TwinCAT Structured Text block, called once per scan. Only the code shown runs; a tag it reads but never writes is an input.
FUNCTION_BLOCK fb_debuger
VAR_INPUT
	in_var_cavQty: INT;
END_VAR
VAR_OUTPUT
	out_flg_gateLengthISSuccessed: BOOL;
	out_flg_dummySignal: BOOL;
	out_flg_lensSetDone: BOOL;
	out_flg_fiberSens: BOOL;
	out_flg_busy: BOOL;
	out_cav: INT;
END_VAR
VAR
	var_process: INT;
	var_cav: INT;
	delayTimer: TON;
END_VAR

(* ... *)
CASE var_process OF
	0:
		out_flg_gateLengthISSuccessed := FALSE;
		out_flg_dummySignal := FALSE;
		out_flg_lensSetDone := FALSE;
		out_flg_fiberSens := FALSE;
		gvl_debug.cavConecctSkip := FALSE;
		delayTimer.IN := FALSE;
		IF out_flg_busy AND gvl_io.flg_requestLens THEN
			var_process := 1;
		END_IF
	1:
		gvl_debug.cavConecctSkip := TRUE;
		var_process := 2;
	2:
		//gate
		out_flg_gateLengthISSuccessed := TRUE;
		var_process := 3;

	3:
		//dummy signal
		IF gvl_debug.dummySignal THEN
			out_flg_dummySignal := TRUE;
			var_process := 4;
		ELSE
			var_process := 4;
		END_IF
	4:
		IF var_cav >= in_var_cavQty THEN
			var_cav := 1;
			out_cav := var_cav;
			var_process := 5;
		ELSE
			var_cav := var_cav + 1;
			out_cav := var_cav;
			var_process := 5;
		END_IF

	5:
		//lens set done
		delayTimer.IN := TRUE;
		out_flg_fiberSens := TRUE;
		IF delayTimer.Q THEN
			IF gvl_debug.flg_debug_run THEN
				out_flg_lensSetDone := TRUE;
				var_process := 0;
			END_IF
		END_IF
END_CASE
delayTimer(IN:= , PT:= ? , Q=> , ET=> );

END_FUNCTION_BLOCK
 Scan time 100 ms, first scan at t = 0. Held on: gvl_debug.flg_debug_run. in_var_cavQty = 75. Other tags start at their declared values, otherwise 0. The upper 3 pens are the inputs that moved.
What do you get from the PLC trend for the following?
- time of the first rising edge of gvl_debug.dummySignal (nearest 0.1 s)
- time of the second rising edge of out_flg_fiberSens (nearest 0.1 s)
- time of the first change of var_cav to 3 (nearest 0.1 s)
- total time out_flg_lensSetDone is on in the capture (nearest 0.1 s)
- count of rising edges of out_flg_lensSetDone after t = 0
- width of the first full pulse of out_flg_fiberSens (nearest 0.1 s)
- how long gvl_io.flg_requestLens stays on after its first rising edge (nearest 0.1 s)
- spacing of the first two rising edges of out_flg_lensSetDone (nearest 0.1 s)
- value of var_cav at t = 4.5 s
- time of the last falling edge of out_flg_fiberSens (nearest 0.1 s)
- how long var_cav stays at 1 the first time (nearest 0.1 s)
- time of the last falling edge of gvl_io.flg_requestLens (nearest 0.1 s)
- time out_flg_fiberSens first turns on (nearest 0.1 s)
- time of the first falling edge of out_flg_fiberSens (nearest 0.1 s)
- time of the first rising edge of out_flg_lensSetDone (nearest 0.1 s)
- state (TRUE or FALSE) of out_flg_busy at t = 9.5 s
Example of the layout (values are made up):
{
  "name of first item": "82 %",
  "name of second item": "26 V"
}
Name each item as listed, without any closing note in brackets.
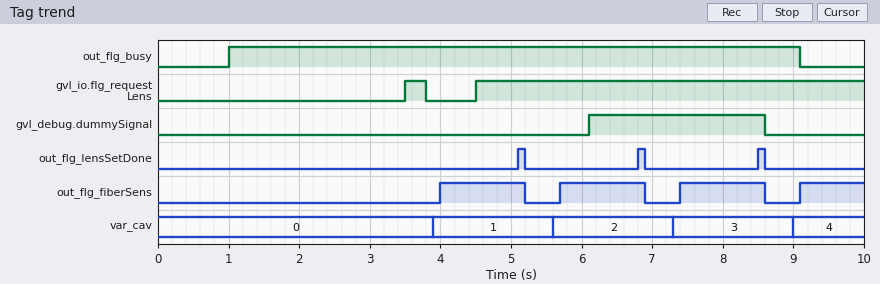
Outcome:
{
  "time of the first rising edge of gvl_debug.dummySignal": "6.1 s",
  "time of the second rising edge of out_flg_fiberSens": "5.7 s",
  "time of the first change of var_cav to 3": "7.3 s",
  "total time out_flg_lensSetDone is on in the capture": "0.3 s",
  "count of rising edges of out_flg_lensSetDone after t = 0": "3",
  "width of the first full pulse of out_flg_fiberSens": "1.2 s",
  "how long gvl_io.flg_requestLens stays on after its first rising edge": "0.3 s",
  "spacing of the first two rising edges of out_flg_lensSetDone": "1.7 s",
  "value of var_cav at t = 4.5 s": "1",
  "time of the last falling edge of out_flg_fiberSens": "8.6 s",
  "how long var_cav stays at 1 the first time": "1.7 s",
  "time of the last falling edge of gvl_io.flg_requestLens": "3.8 s",
  "time out_flg_fiberSens first turns on": "4.0 s",
  "time of the first falling edge of out_flg_fiberSens": "5.2 s",
  "time of the first rising edge of out_flg_lensSetDone": "5.1 s",
  "state (TRUE or FALSE) of out_flg_busy at t = 9.5 s": "FALSE"
}
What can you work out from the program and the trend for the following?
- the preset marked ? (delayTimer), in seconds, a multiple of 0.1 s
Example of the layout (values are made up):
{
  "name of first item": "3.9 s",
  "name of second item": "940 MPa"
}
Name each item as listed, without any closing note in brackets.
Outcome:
{
  "the preset marked ? (delayTimer), in seconds, a multiple of 0.1 s": "1.0 s"
}
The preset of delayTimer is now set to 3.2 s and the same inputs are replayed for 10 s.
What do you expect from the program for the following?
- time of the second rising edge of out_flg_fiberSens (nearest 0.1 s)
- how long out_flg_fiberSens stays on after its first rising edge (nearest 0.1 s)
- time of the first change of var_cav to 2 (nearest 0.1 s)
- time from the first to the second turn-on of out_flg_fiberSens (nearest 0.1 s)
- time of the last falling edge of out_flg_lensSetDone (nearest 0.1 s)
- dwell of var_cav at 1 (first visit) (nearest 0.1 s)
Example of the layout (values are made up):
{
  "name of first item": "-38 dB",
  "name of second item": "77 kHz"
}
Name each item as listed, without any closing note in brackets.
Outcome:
{
  "time of the second rising edge of out_flg_fiberSens": "7.9 s",
  "how long out_flg_fiberSens stays on after its first rising edge": "3.4 s",
  "time of the first change of var_cav to 2": "7.8 s",
  "time from the first to the second turn-on of out_flg_fiberSens": "3.9 s",
  "time of the last falling edge of out_flg_lensSetDone": "7.4 s",
  "dwell of var_cav at 1 (first visit)": "3.9 s"
}
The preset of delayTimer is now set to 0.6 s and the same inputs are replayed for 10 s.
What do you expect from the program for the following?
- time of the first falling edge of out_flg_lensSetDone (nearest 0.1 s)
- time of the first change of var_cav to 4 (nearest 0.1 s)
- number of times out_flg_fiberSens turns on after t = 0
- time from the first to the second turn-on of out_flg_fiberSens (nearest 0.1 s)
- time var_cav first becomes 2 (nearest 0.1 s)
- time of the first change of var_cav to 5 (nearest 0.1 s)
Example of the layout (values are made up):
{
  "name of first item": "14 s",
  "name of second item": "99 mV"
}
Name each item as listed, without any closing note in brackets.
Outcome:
{
  "time of the first falling edge of out_flg_lensSetDone": "4.8 s",
  "time of the first change of var_cav to 4": "7.8 s",
  "number of times out_flg_fiberSens turns on after t = 0": "5",
  "time from the first to the second turn-on of out_flg_fiberSens": "1.3 s",
  "time var_cav first becomes 2": "5.2 s",
  "time of the first change of var_cav to 5": "9.1 s"
}
